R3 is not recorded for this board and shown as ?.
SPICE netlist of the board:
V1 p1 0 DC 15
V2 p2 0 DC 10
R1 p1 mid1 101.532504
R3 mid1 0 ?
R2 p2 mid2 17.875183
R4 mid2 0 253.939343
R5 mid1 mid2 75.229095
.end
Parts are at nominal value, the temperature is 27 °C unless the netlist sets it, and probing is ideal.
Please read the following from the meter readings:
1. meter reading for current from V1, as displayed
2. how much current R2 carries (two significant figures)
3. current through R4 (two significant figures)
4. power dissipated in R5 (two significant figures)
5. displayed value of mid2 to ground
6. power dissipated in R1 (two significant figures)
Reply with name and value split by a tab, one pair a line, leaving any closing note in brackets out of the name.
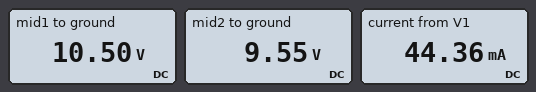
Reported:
meter reading for current from V1, as displayed	44.36 mA
how much current R2 carries	25 mA
current through R4	38 mA
power dissipated in R5	12 mW
displayed value of mid2 to ground	9.55 V
power dissipated in R1	200 mW
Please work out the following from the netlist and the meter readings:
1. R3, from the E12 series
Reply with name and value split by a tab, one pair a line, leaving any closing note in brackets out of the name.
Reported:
R3, from the E12 series	330 Ω
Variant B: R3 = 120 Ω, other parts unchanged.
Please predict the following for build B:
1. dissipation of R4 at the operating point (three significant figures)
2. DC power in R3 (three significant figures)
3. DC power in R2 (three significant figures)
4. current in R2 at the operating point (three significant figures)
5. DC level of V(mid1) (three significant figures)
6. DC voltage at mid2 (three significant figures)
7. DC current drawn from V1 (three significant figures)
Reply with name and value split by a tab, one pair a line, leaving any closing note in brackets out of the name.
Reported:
dissipation of R4 at the operating point	334 mW
DC power in R3	614 mW
DC power in R2	35.4 mW
current in R2 at the operating point	44.5 mA
DC level of V(mid1)	8.58 V
DC voltage at mid2	9.20 V
DC current drawn from V1	63.2 mA
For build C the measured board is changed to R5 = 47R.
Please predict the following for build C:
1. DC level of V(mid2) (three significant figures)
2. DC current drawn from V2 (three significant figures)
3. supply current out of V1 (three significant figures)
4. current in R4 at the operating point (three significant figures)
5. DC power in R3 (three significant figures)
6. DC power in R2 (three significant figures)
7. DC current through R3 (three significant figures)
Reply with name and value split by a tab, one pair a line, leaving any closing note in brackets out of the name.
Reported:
DC level of V(mid2)	9.59 V
DC current drawn from V2	22.7 mA
supply current out of V1	46.3 mA
current in R4 at the operating point	37.8 mA
DC power in R3	322 mW
DC power in R2	9.23 mW
DC current through R3	31.2 mA
